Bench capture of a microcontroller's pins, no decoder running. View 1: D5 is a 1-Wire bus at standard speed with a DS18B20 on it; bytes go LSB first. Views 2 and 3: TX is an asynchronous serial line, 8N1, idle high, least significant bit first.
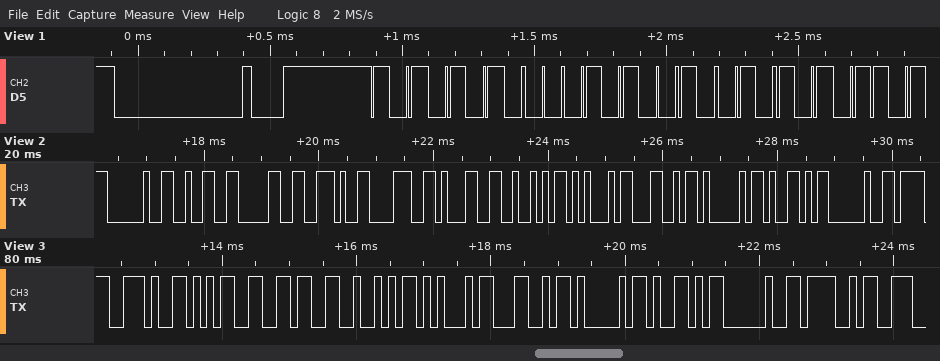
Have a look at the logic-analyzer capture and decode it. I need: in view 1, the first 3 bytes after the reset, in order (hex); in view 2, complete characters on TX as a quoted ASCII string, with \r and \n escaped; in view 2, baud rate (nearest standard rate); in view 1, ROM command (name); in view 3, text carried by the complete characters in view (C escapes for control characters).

55 28 A9
" 20.81RELAY "
9600 baud
Match ROM
".56RELAY O"
